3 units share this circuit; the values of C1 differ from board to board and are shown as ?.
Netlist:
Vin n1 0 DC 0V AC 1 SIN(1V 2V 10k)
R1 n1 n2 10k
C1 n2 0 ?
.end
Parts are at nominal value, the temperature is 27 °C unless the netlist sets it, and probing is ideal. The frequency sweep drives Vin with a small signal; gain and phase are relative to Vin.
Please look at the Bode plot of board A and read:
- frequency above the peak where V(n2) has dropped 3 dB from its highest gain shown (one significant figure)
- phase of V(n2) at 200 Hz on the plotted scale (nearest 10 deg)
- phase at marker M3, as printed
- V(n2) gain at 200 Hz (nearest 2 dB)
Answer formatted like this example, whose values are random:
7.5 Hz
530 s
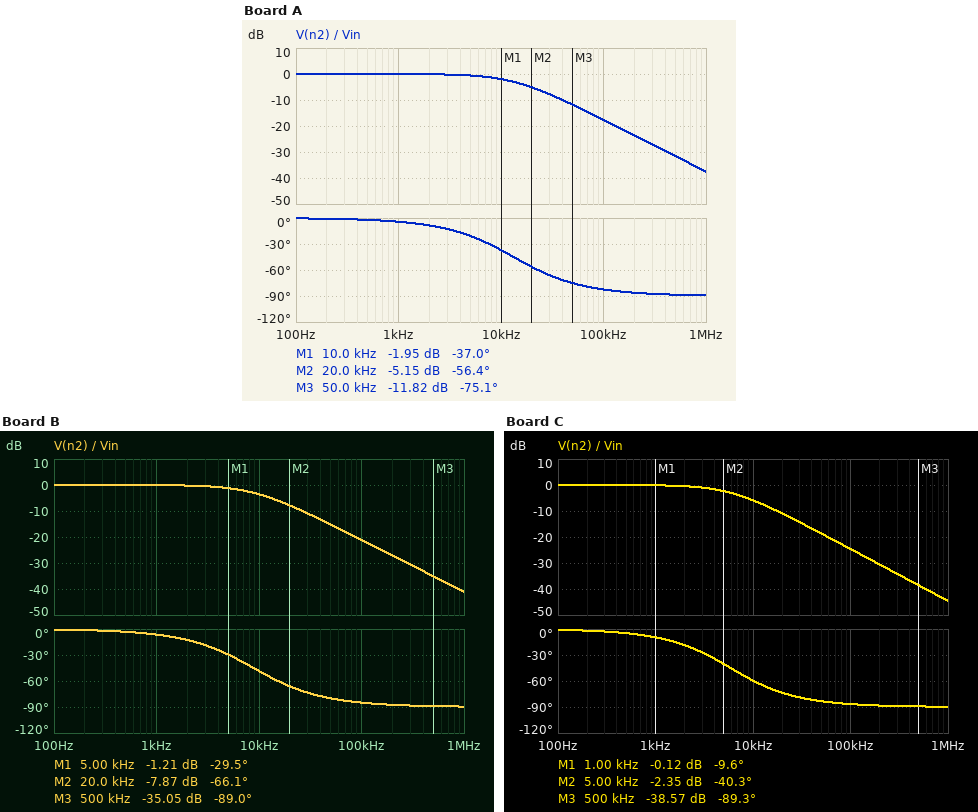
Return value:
10 kHz
0 deg
-75.1 deg
0 dB
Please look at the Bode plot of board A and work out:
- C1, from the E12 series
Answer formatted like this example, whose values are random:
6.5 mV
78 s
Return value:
1.2 nF
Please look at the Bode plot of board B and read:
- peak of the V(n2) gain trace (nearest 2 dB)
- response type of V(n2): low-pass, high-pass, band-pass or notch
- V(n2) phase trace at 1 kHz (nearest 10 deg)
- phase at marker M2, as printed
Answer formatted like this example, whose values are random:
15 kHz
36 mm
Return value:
0 dB
low-pass
-10 deg
-66.1 deg
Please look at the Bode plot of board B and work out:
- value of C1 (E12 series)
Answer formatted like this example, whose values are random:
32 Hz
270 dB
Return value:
1.8 nF
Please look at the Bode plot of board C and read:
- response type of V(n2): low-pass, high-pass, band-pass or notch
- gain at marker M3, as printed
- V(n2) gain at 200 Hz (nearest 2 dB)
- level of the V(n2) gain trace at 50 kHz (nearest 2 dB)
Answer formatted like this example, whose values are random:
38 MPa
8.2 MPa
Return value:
low-pass
-38.57 dB
0 dB
-18 dB
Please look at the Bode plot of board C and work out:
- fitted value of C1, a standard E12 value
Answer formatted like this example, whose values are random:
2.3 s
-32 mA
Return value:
2.7 nF
